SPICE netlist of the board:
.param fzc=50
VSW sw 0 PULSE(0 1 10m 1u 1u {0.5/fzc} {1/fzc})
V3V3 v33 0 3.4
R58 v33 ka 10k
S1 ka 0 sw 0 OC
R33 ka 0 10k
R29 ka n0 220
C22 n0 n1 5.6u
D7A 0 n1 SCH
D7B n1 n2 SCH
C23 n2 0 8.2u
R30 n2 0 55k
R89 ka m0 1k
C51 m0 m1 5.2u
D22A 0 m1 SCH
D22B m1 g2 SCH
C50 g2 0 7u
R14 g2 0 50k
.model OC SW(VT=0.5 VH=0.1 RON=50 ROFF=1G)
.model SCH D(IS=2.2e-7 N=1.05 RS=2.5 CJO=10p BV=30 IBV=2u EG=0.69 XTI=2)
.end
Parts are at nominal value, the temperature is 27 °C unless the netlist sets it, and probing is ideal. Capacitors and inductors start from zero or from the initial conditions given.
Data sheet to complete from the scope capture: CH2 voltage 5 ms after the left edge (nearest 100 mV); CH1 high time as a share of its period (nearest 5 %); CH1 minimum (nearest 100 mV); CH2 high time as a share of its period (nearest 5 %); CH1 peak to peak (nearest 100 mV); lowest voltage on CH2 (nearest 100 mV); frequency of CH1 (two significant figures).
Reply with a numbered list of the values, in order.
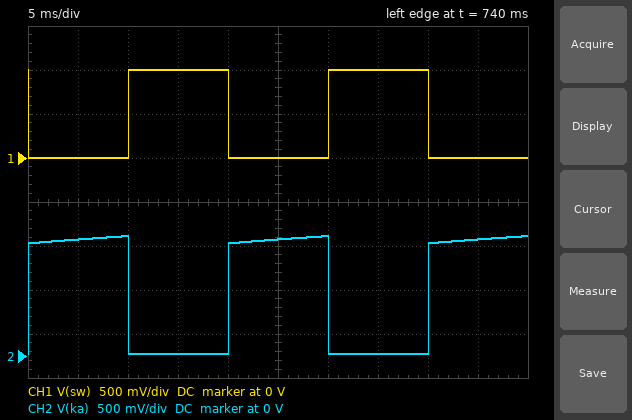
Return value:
1. 1.3 V
2. 50 %
3. 0 V
4. 50 %
5. 1.0 V
6. 0 V
7. 50 Hz
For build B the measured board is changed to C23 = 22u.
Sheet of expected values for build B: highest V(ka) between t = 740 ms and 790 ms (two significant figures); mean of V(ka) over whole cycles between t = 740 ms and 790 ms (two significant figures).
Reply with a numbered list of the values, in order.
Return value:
1. 1.3 V
2. 650 mV
